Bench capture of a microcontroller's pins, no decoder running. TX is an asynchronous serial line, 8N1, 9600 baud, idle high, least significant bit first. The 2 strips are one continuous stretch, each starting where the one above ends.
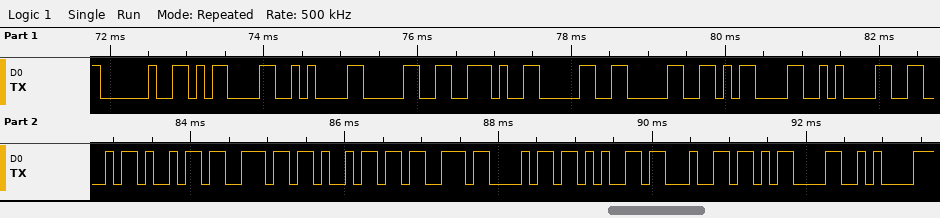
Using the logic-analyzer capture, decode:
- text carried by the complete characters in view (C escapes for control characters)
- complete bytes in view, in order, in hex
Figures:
" \r\n0.00\r\nFinished\r\n"
20 0D 0A 30 2E 30 30 0D 0A 46 69 6E 69 73 68 65 64 0D 0A
